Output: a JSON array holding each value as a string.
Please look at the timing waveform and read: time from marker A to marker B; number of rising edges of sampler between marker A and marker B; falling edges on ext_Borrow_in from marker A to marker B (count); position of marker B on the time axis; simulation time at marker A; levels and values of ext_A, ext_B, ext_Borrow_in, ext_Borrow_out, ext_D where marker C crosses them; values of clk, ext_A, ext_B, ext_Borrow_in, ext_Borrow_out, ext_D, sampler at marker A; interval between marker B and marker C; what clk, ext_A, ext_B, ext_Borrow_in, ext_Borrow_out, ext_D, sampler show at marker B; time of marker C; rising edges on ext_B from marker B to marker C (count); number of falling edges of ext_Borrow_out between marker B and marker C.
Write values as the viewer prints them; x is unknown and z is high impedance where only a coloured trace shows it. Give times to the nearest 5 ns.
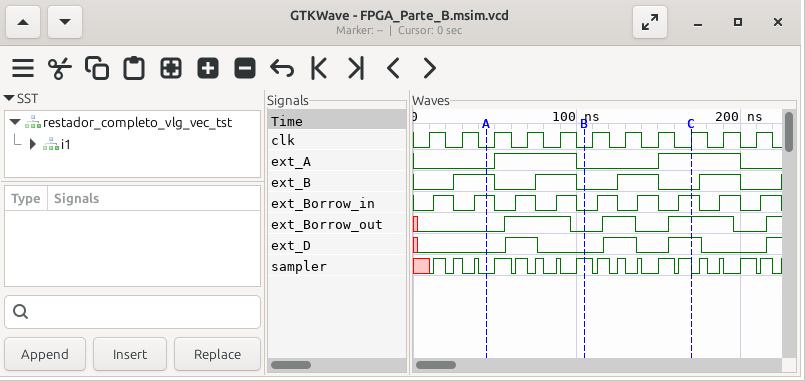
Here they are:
["60 ns", "5", "3", "105 ns", "45 ns", "ext_A=1, ext_B=0, ext_Borrow_in=1, ext_Borrow_out=1, ext_D=1", "clk=0, ext_A=0, ext_B=1, ext_Borrow_in=1, ext_Borrow_out=0, ext_D=0, sampler=0", "65 ns", "clk=0, ext_A=0, ext_B=0, ext_Borrow_in=0, ext_Borrow_out=0, ext_D=0, sampler=1", "170 ns", "1", "1"]
